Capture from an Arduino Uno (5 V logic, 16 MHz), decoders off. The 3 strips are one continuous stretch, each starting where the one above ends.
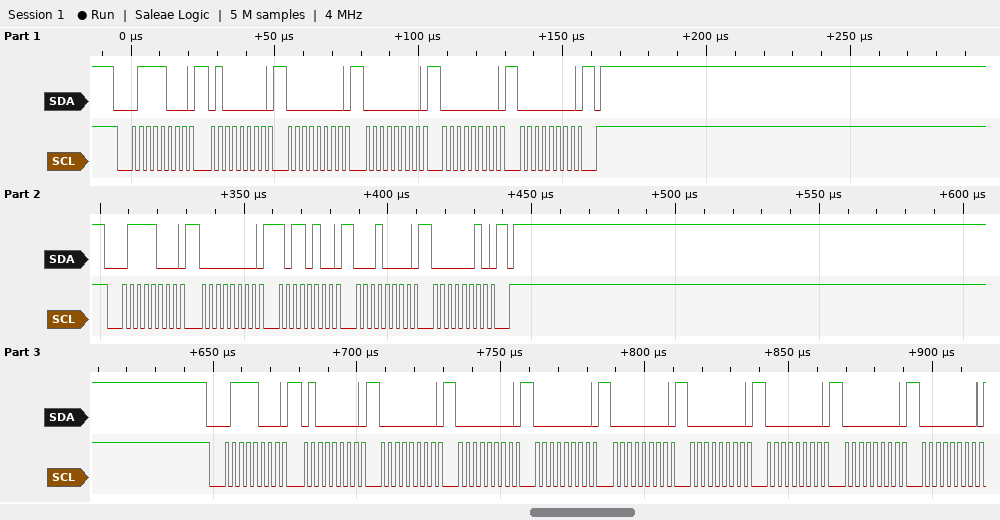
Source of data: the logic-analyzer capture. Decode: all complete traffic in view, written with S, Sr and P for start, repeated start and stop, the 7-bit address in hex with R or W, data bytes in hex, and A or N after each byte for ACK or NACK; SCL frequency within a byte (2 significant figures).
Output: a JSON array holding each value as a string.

["S 3CW A 40 A 00 A 00 A 00 A 00 A P S 3CW A 00 A B4 A 10 A 02 A P S 3CW A 40 A 00 A 00 A 00 A 00 A 00 A 00 A 00 A 00 A", "400 kHz"]
